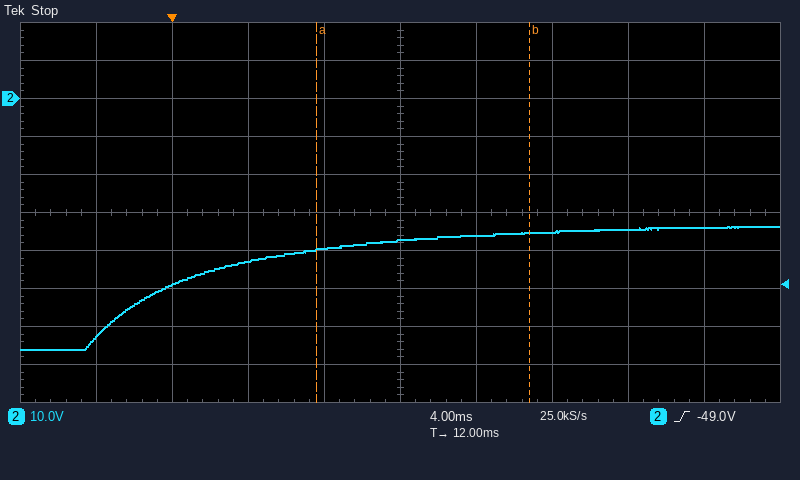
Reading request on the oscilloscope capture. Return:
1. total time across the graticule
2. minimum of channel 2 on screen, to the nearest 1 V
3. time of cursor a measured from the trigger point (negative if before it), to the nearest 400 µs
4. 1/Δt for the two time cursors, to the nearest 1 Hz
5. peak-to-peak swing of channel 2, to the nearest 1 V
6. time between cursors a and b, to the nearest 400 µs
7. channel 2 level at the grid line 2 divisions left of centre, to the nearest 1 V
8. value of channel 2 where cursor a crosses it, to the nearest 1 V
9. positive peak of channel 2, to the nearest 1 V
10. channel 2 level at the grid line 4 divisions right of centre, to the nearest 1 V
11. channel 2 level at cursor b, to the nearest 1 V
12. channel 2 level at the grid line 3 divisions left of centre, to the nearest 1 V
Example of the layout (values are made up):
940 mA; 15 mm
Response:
40 ms; -66 V; +7.6 ms; 89 Hz; 32 V; 11.2 ms; -43 V; -40 V; -34 V; -34 V; -35 V; -49 V
